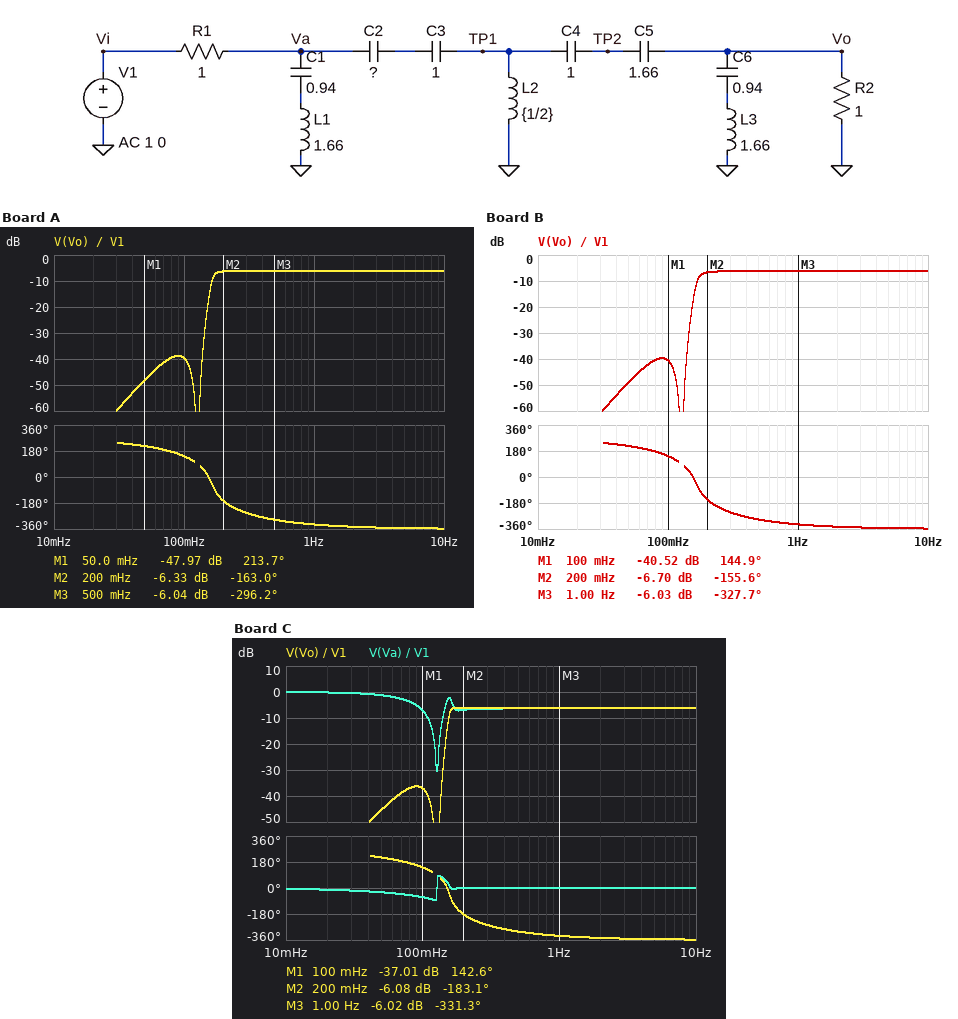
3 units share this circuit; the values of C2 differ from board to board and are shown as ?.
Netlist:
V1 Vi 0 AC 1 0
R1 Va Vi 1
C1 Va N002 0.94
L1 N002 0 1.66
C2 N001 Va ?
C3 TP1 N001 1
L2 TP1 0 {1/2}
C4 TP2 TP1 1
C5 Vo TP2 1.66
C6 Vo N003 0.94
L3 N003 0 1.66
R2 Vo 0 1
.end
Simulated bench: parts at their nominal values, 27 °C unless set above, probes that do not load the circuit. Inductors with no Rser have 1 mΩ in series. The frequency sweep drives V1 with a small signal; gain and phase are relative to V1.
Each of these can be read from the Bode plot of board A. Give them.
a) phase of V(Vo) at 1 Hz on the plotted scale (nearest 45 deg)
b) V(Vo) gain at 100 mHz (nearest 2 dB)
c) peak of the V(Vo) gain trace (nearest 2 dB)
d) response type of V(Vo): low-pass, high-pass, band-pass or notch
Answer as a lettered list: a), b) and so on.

a) -315 deg
b) -40 dB
c) -6 dB
d) high-pass
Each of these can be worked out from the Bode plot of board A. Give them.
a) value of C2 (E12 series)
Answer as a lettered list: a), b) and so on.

a) 1 F
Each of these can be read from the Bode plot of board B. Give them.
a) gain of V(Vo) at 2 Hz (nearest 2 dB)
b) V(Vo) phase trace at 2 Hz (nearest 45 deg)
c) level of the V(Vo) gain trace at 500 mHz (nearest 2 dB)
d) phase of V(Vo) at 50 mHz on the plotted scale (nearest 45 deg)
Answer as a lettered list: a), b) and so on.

a) -6 dB
b) -360 deg
c) -6 dB
d) 225 deg
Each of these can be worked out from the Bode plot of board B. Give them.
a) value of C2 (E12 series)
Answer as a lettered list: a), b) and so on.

a) 820 mF
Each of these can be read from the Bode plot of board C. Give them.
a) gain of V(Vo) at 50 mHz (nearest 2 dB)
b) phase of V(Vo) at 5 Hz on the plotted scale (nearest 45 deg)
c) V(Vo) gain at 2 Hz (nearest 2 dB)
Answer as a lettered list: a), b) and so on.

a) -46 dB
b) -360 deg
c) -6 dB
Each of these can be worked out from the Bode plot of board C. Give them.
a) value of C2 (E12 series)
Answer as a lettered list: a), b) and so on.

a) 2.2 F
